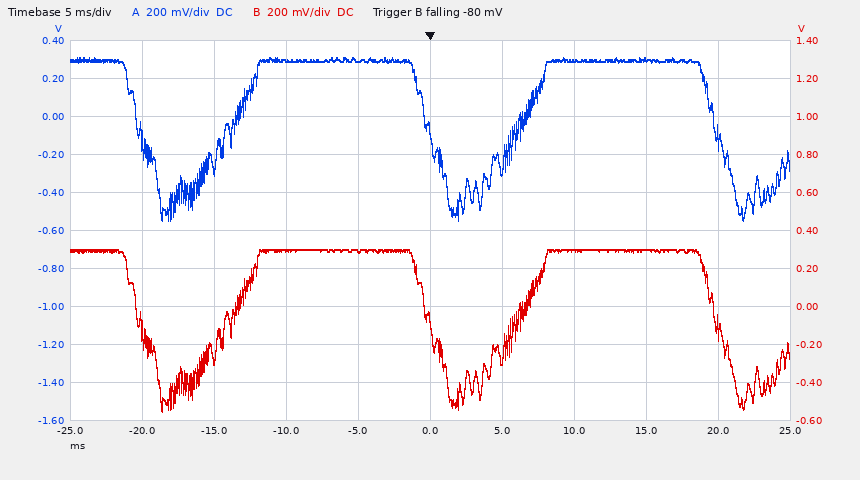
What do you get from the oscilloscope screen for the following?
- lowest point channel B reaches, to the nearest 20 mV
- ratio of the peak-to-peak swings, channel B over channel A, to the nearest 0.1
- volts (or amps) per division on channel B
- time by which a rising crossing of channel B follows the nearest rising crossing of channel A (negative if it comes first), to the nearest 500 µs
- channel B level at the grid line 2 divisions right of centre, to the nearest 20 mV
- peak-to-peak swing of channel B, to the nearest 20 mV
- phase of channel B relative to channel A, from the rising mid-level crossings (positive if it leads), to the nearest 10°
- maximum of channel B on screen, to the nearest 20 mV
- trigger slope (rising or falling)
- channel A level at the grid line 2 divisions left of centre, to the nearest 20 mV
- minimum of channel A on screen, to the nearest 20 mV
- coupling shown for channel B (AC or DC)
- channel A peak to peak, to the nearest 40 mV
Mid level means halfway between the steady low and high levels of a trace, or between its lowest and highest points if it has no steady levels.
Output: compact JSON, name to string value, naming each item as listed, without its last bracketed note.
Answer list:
{"lowest point channel B reaches, to the nearest 20 mV": "-560 mV", "ratio of the peak-to-peak swings, channel B over channel A, to the nearest 0.1": "1.0", "volts (or amps) per division on channel B": "200 mV", "time by which a rising crossing of channel B follows the nearest rising crossing of channel A (negative if it comes first), to the nearest 500 µs": "0.0 ms", "channel B level at the grid line 2 divisions right of centre, to the nearest 20 mV": "300 mV", "peak-to-peak swing of channel B, to the nearest 20 mV": "860 mV", "phase of channel B relative to channel A, from the rising mid-level crossings (positive if it leads), to the nearest 10°": "0°", "maximum of channel B on screen, to the nearest 20 mV": "300 mV", "trigger slope": "falling", "channel A level at the grid line 2 divisions left of centre, to the nearest 20 mV": "300 mV", "minimum of channel A on screen, to the nearest 20 mV": "-540 mV", "coupling shown for channel B": "DC", "channel A peak to peak, to the nearest 40 mV": "840 mV"}
